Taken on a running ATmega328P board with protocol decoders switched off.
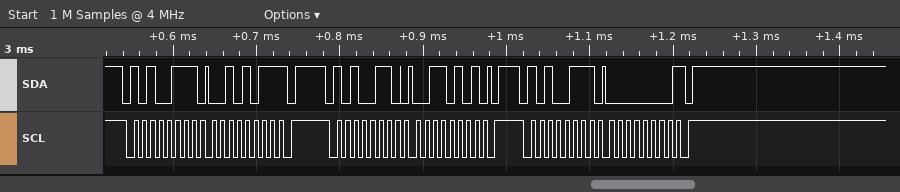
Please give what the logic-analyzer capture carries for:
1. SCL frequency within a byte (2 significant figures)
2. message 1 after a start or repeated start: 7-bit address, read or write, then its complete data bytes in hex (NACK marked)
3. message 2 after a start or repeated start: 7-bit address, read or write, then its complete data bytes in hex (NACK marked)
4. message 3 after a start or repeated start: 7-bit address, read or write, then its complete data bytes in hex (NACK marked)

100 kHz
0x53 read: 2B NACK
0x53 write: 35
0x53 read: 00 NACK
